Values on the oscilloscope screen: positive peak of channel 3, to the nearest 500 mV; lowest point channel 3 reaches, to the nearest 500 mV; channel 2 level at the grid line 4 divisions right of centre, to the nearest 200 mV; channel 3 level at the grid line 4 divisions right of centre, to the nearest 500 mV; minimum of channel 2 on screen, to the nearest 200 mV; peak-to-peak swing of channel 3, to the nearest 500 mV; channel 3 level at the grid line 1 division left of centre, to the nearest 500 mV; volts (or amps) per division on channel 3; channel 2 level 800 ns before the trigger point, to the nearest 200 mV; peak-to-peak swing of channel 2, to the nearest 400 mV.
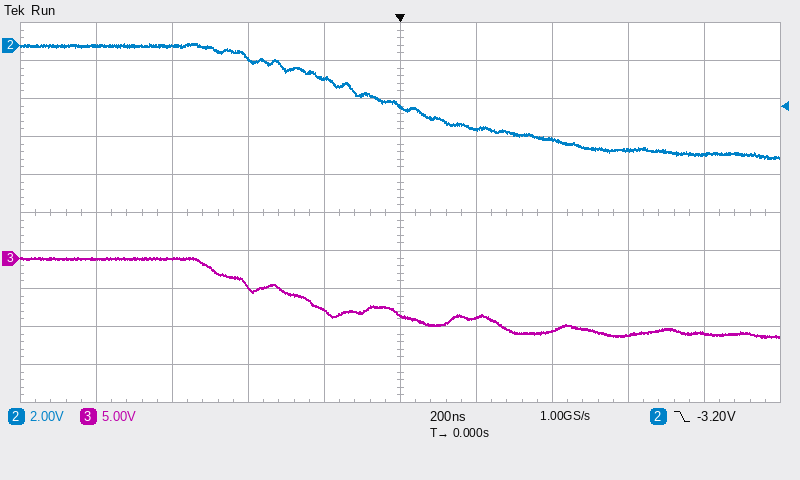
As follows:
0.0 V
-10.5 V
-5.8 V
-10.0 V
-6.0 V
10.5 V
-7.0 V
5 V
0.0 V
6.0 V
